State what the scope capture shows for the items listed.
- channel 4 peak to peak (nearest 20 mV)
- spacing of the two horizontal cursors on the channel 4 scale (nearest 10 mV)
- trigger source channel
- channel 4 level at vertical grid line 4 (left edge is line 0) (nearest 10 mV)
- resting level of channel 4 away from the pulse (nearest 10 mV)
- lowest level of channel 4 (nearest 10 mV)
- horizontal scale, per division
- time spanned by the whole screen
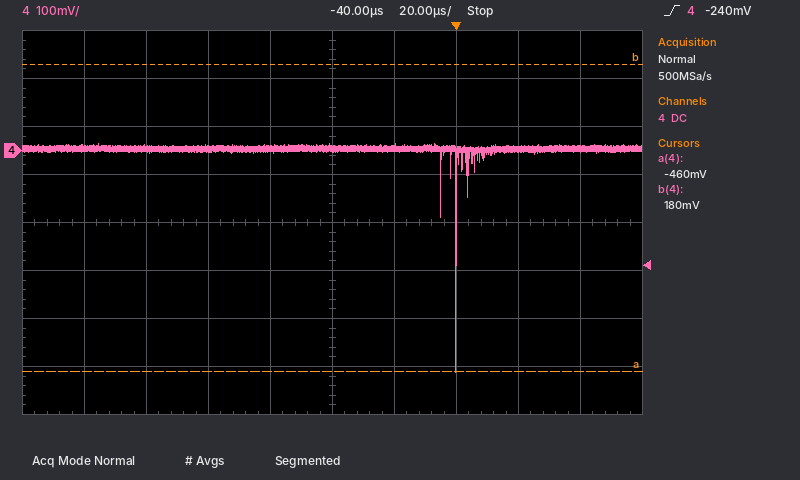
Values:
480 mV
640 mV
channel 4
0 mV
0 mV
-460 mV
20 µs
200 µs
